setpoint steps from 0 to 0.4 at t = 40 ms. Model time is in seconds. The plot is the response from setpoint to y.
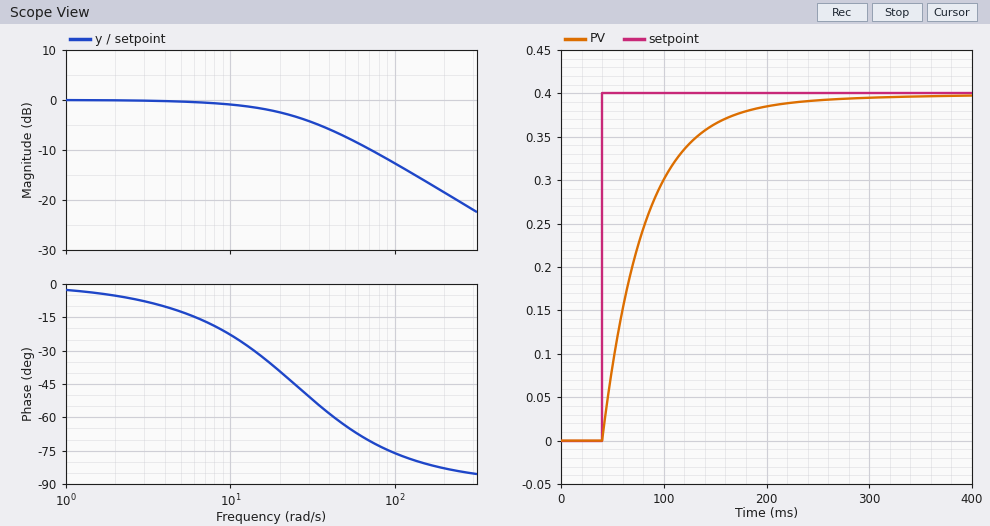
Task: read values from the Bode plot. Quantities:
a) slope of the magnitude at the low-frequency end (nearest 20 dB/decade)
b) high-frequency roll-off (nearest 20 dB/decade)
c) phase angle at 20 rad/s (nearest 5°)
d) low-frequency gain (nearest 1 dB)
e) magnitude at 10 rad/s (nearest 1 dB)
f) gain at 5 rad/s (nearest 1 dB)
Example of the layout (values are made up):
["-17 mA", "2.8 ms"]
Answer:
["0 dB/decade", "-20 dB/decade", "-40°", "0 dB", "-1 dB", "0 dB"]
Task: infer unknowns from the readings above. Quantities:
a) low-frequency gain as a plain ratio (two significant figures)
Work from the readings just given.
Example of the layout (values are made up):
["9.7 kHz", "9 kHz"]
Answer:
["1.0"]
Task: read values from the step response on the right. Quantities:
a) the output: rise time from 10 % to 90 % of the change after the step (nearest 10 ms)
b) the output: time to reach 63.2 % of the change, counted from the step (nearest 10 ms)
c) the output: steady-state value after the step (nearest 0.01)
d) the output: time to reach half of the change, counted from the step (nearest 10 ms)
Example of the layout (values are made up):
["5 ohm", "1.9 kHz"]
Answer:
["100 ms", "40 ms", "0.40", "30 ms"]
